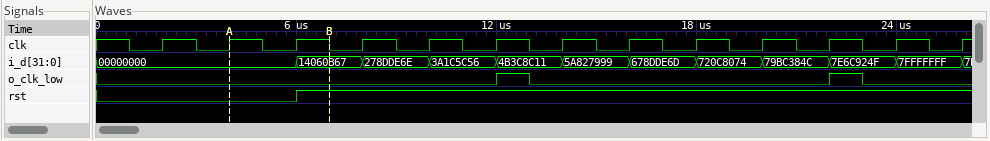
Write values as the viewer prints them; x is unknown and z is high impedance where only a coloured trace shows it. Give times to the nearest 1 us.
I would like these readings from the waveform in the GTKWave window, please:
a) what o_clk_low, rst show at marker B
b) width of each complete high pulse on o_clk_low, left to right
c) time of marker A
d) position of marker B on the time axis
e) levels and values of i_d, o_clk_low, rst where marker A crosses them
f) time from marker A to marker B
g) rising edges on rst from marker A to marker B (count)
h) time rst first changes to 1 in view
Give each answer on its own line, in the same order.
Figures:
o_clk_low=0, rst=1
1 us, 1 us
4 us
7 us
i_d=00000000, o_clk_low=0, rst=0
3 us
1
6 us
